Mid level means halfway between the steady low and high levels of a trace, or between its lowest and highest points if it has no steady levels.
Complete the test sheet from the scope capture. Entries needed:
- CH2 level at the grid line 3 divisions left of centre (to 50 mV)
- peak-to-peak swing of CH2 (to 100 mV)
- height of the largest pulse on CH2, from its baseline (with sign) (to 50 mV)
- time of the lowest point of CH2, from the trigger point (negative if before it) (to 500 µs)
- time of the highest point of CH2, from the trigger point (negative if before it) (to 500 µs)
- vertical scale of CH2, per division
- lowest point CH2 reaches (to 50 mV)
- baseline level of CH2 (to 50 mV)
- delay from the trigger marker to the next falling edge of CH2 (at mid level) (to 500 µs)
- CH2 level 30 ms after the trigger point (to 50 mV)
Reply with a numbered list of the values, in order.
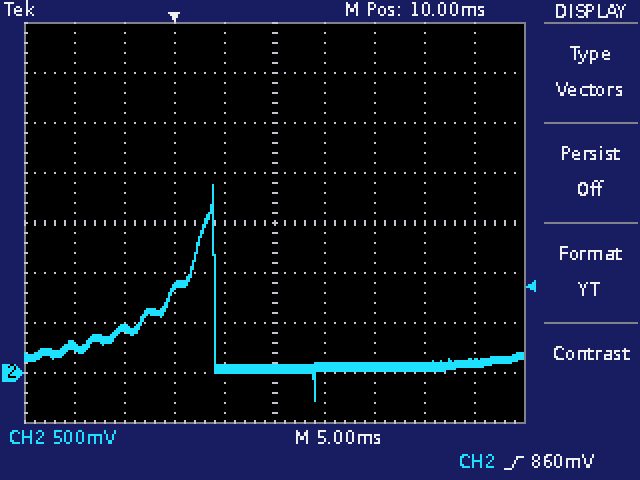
1. 450 mV
2. 2.20 V
3. +1.80 V
4. +14.0 ms
5. +4.0 ms
6. 500 mV
7. -300 mV
8. 50 mV
9. 4.0 ms
10. 100 mV
